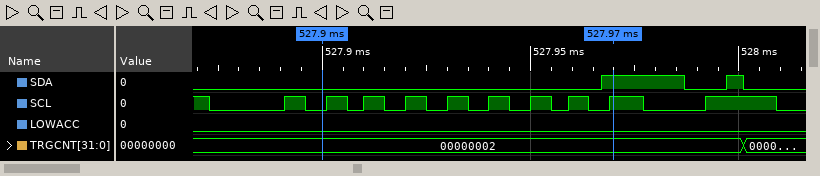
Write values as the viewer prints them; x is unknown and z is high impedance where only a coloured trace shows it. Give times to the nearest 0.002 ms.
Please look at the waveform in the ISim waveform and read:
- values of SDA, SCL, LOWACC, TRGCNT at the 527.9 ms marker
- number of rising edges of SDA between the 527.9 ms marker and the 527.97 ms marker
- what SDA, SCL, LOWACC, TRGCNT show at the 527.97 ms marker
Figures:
SDA=0, SCL=0, LOWACC=0, TRGCNT=00000002
1
SDA=1, SCL=1, LOWACC=0, TRGCNT=00000002
